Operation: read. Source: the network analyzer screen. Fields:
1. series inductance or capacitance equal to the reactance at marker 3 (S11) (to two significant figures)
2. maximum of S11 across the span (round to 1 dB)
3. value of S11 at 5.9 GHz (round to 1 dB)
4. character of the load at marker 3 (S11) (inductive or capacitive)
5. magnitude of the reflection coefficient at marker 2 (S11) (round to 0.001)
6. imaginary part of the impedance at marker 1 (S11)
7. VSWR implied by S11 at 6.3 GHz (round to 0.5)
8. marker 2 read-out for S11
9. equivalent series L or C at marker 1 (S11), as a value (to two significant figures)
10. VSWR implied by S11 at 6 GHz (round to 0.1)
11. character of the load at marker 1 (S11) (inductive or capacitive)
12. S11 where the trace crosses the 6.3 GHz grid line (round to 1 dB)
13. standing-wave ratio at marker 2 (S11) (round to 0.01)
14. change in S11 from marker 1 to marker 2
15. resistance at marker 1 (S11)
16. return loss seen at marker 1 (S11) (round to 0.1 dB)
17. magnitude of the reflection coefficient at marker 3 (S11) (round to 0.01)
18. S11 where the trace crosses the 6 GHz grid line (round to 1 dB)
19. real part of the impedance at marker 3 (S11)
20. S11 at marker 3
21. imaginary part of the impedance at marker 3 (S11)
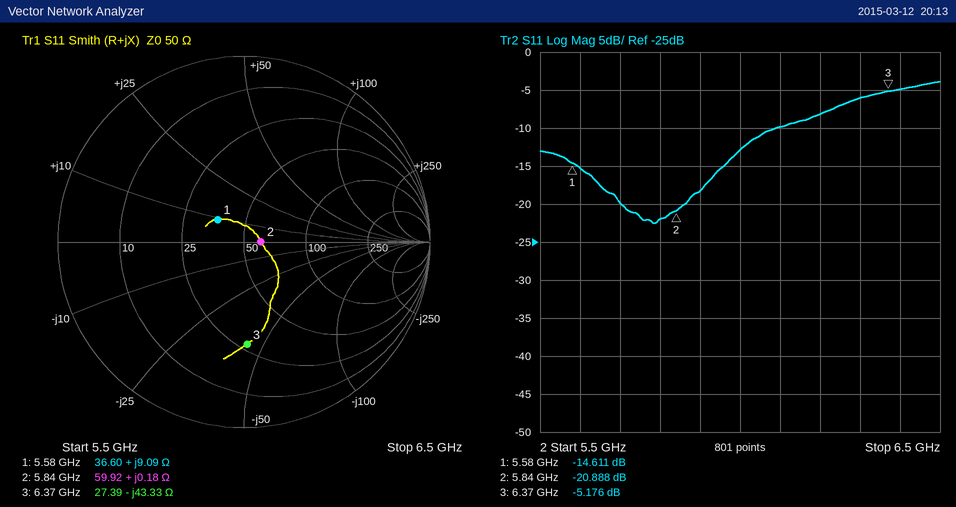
580 fF
-4 dB
-18 dB
capacitive
0.090
+9.09 Ω
3.0
-20.888 dB
260 pH
1.6
inductive
-6 dB
1.20
-6.277 dB
36.60 Ω
14.6 dB
0.55
-13 dB
27.39 Ω
-5.176 dB
-43.33 Ω
